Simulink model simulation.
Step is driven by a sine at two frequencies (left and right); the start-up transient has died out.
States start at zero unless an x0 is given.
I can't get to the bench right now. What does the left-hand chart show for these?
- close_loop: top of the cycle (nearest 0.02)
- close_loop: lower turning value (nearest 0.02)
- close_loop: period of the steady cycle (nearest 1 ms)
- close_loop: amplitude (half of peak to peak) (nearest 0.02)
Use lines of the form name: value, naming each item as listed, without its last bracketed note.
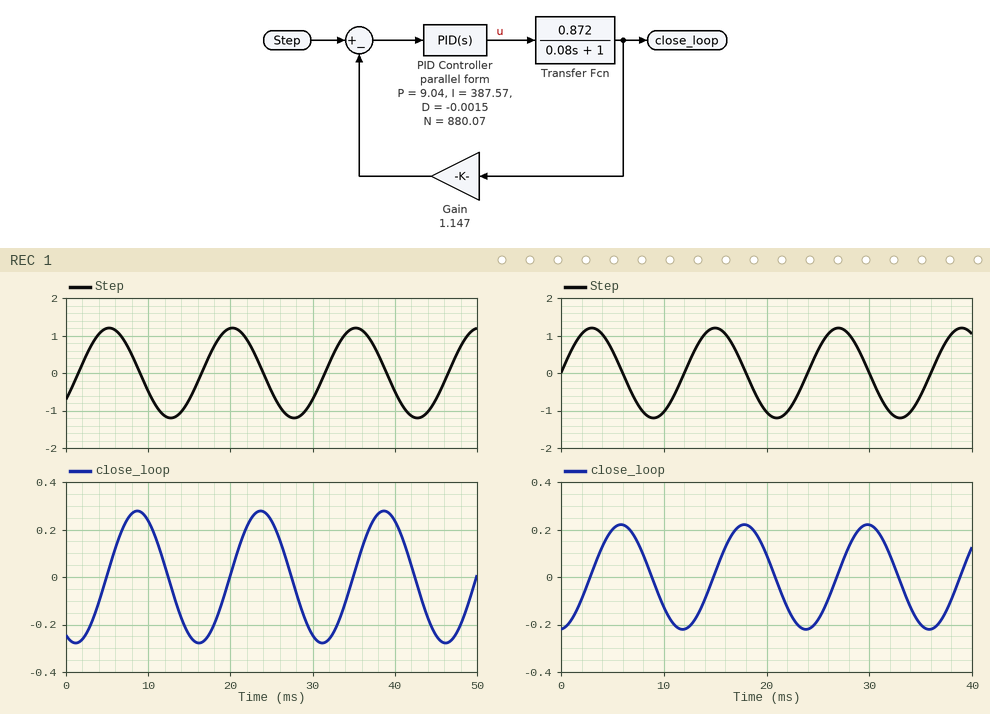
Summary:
close_loop: top of the cycle: 0.28
close_loop: lower turning value: -0.28
close_loop: period of the steady cycle: 15 ms
close_loop: amplitude (half of peak to peak): 0.28
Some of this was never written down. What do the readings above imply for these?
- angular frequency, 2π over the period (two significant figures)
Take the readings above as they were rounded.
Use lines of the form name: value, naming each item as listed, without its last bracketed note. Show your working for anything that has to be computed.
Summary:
angular frequency, 2π over the period: 2π / 15 = 0.42 rad/ms
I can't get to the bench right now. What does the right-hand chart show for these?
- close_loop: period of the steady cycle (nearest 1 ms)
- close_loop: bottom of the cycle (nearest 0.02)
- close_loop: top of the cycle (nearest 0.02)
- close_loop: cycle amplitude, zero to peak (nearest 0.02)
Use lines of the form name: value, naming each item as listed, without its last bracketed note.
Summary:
close_loop: period of the steady cycle: 12 ms
close_loop: bottom of the cycle: -0.22
close_loop: top of the cycle: 0.22
close_loop: cycle amplitude, zero to peak: 0.22
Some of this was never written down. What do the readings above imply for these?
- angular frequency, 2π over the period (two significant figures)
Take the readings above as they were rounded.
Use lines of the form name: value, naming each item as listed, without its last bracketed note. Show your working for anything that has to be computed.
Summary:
angular frequency, 2π over the period: 2π / 12 = 0.52 rad/ms
